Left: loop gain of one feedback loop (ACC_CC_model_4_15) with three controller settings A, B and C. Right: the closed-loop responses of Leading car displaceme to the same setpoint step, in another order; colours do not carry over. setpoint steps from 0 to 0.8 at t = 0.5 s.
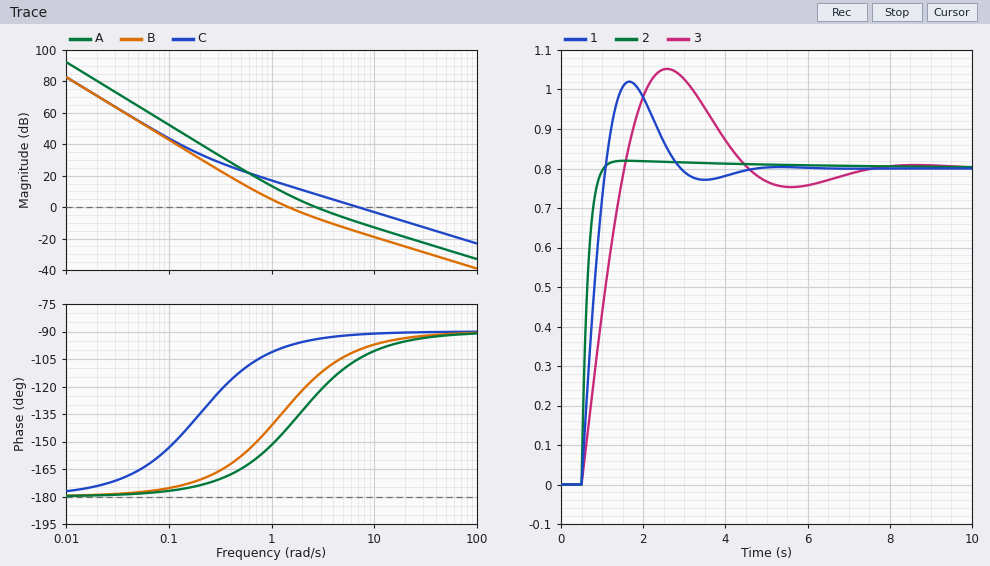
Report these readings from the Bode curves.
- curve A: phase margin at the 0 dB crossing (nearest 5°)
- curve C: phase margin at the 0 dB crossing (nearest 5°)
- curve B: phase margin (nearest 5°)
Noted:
55°
90°
50°
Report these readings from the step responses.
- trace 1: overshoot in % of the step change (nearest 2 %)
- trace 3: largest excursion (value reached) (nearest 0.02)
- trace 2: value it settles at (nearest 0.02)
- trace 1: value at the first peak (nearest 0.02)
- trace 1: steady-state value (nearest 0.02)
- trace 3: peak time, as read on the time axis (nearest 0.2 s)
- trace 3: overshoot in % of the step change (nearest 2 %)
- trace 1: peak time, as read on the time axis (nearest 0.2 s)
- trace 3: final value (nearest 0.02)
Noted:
28 %
1.06
0.80
1.02
0.80
2.6 s
32 %
1.6 s
0.80
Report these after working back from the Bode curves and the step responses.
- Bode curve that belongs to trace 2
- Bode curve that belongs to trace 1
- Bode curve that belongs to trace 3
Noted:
C
A
B
